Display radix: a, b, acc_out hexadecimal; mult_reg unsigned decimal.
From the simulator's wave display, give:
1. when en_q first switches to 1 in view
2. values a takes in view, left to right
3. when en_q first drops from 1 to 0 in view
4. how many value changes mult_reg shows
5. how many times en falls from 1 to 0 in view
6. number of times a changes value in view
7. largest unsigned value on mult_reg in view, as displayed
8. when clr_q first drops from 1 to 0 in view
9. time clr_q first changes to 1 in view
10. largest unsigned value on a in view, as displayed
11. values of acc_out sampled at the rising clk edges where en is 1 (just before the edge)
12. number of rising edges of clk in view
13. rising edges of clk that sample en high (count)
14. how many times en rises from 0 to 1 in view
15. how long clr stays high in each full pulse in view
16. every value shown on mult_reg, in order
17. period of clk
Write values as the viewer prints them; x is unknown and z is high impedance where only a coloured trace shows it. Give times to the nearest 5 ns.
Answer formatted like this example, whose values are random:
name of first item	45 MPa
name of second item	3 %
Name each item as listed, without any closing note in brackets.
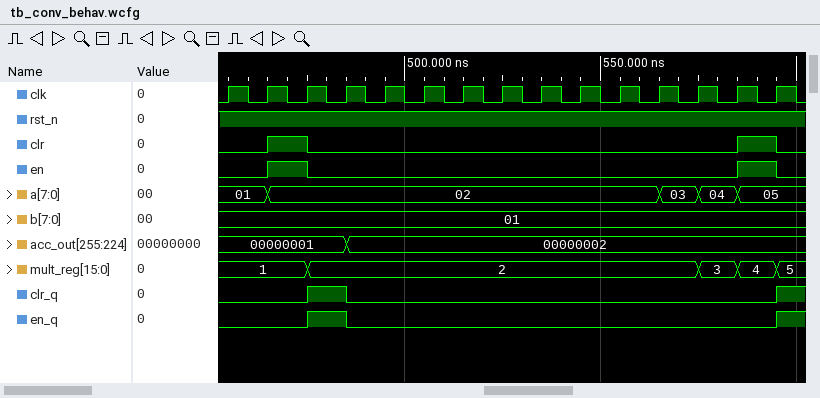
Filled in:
when en_q first switches to 1 in view	475 ns
values a takes in view, left to right	01, 02, 03, 04, 05
when en_q first drops from 1 to 0 in view	485 ns
how many value changes mult_reg shows	4
how many times en falls from 1 to 0 in view	2
number of times a changes value in view	4
largest unsigned value on mult_reg in view, as displayed	5
when clr_q first drops from 1 to 0 in view	485 ns
time clr_q first changes to 1 in view	475 ns
largest unsigned value on a in view, as displayed	05
values of acc_out sampled at the rising clk edges where en is 1	00000001, 00000002
number of rising edges of clk in view	15
rising edges of clk that sample en high	2
how many times en rises from 0 to 1 in view	2
how long clr stays high in each full pulse in view	10 ns, 10 ns
every value shown on mult_reg, in order	1, 2, 3, 4, 5
period of clk	10 ns
